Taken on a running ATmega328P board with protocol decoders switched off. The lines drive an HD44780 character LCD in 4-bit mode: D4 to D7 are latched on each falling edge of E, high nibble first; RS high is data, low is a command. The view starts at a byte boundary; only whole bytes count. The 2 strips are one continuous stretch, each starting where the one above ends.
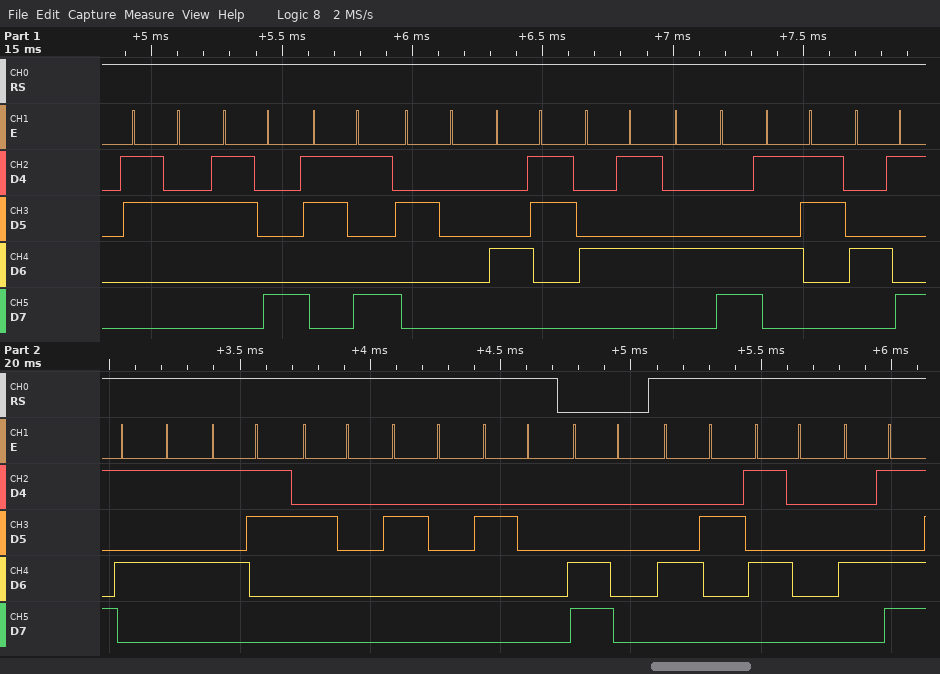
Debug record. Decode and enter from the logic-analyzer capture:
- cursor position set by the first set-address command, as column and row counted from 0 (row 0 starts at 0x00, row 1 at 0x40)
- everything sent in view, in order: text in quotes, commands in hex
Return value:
column 0, row 1
"289 CELSIUS   " 0xC0 "BPM"
